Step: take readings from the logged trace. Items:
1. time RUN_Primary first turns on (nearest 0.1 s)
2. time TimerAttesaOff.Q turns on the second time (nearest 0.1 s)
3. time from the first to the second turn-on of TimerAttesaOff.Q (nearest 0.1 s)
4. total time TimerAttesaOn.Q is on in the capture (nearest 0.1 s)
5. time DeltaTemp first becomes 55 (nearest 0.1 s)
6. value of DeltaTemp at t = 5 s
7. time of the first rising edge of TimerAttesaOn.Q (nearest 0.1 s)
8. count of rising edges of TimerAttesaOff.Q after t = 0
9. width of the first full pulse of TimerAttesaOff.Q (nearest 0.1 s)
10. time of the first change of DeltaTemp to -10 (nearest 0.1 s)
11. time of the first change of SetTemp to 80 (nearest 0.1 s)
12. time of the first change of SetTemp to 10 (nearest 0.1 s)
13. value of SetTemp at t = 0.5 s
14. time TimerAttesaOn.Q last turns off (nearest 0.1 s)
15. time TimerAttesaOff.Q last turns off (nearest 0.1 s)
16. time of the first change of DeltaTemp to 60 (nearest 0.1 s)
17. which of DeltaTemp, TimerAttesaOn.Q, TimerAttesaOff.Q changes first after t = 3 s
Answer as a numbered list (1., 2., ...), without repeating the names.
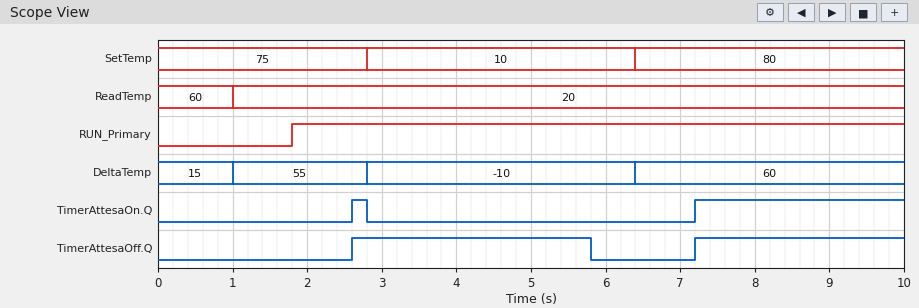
1. 1.8 s
2. 7.2 s
3. 4.6 s
4. 3.0 s
5. 1.0 s
6. -10
7. 2.6 s
8. 2
9. 3.2 s
10. 2.8 s
11. 6.4 s
12. 2.8 s
13. 75
14. 2.8 s
15. 5.8 s
16. 6.4 s
17. TimerAttesaOff.Q
